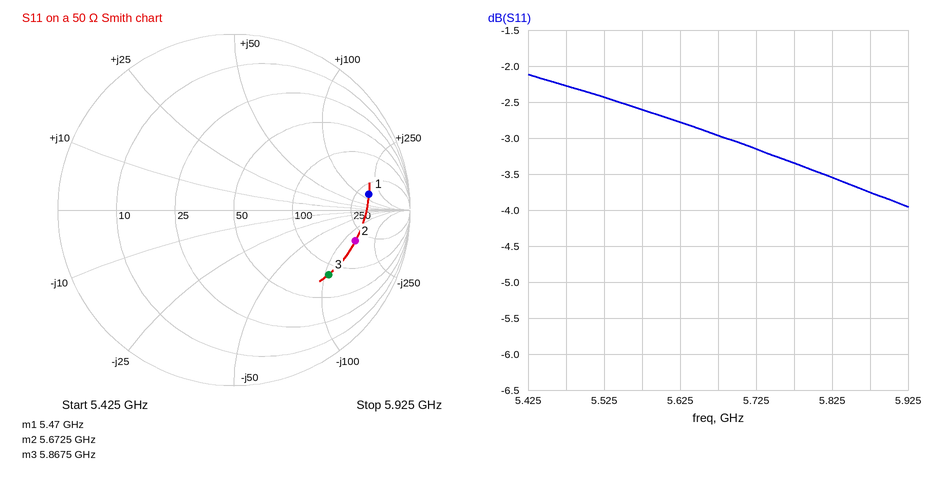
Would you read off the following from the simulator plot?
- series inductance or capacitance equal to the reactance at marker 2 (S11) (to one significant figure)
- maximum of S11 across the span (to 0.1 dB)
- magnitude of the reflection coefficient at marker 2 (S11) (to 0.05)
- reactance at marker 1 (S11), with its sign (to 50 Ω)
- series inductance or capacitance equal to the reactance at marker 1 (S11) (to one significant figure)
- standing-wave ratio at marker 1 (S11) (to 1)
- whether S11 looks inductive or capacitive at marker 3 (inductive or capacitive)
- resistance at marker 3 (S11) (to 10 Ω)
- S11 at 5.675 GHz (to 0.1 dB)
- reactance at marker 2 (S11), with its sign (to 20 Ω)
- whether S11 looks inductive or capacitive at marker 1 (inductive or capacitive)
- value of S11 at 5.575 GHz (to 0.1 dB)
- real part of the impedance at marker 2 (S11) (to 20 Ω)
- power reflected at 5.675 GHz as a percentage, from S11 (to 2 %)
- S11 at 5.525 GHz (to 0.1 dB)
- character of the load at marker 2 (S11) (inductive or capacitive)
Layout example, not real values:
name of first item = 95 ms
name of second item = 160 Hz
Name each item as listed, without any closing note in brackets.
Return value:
series inductance or capacitance equal to the reactance at marker 2 (S11) = 200 fF
maximum of S11 across the span = -2.1 dB
magnitude of the reflection coefficient at marker 2 (S11) = 0.70
reactance at marker 1 (S11), with its sign = +150 Ω
series inductance or capacitance equal to the reactance at marker 1 (S11) = 4 nH
standing-wave ratio at marker 1 (S11) = 8
whether S11 looks inductive or capacitive at marker 3 = capacitive
resistance at marker 3 (S11) = 80 Ω
S11 at 5.675 GHz = -3.0 dB
reactance at marker 2 (S11), with its sign = -140 Ω
whether S11 looks inductive or capacitive at marker 1 = inductive
value of S11 at 5.575 GHz = -2.6 dB
real part of the impedance at marker 2 (S11) = 200 Ω
power reflected at 5.675 GHz as a percentage, from S11 = 50 %
S11 at 5.525 GHz = -2.4 dB
character of the load at marker 2 (S11) = capacitive
